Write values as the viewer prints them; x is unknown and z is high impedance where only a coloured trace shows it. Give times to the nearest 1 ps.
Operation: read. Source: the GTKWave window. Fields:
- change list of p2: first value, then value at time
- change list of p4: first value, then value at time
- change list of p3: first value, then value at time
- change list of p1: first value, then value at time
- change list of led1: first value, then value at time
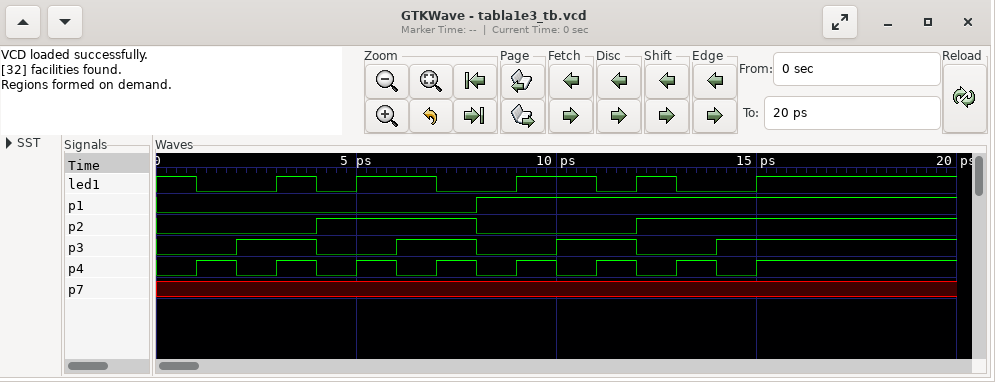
0, 1 at 4 ps, 0 at 8 ps, 1 at 12 ps
0, 1 at 1 ps, 0 at 2 ps, 1 at 3 ps, 0 at 4 ps, 1 at 5 ps, 0 at 6 ps, 1 at 7 ps, 0 at 8 ps, 1 at 9 ps, 0 at 10 ps, 1 at 11 ps, 0 at 12 ps, 1 at 13 ps, 0 at 14 ps, 1 at 15 ps
0, 1 at 2 ps, 0 at 4 ps, 1 at 6 ps, 0 at 8 ps, 1 at 10 ps, 0 at 12 ps, 1 at 14 ps
0, 1 at 8 ps
1, 0 at 1 ps, 1 at 3 ps, 0 at 4 ps, 1 at 5 ps, 0 at 7 ps, 1 at 9 ps, 0 at 11 ps, 1 at 12 ps, 0 at 13 ps, 1 at 15 ps
